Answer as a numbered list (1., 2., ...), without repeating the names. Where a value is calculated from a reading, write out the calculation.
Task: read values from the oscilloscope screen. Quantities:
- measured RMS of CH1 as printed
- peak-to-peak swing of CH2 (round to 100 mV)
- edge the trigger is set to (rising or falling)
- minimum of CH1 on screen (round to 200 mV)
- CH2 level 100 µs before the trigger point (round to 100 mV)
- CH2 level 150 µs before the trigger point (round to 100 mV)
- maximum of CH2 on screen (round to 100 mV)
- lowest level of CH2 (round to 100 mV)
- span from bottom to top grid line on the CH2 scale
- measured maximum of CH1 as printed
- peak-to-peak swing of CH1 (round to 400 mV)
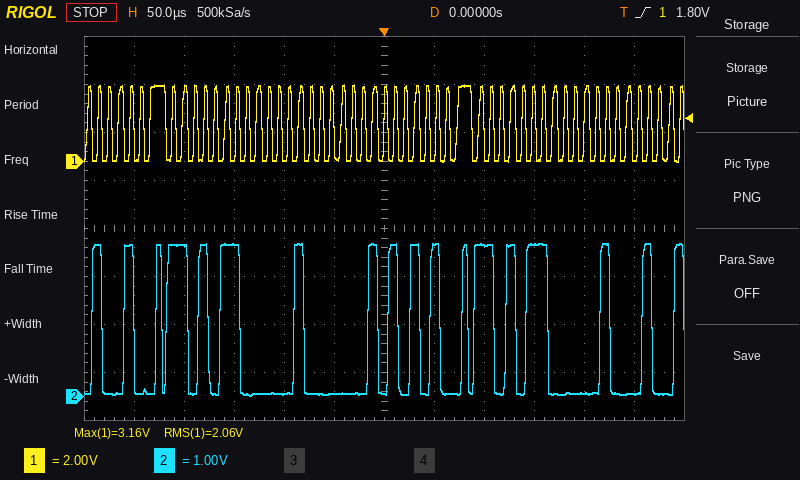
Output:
1. 2.06 V
2. 3.2 V − (0.0 V) = 3.2 V
3. rising
4. 0.0 V
5. 100 mV
6. 3.2 V
7. 3.2 V
8. 0.0 V
9. 8 V
10. 3.16 V
11. 3.2 V
